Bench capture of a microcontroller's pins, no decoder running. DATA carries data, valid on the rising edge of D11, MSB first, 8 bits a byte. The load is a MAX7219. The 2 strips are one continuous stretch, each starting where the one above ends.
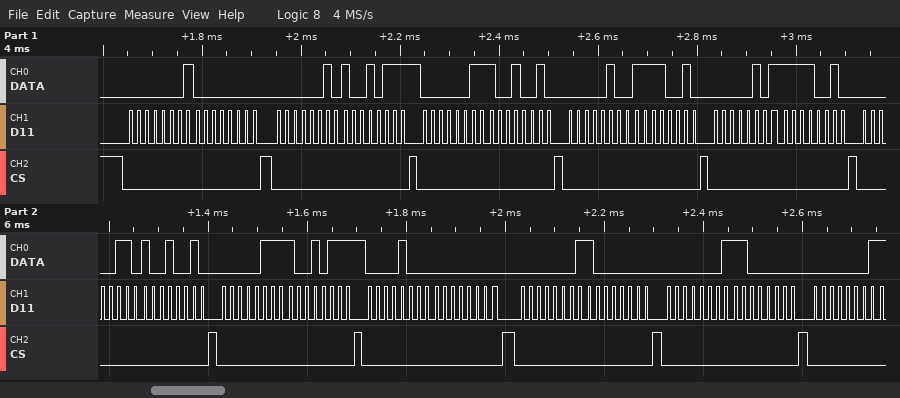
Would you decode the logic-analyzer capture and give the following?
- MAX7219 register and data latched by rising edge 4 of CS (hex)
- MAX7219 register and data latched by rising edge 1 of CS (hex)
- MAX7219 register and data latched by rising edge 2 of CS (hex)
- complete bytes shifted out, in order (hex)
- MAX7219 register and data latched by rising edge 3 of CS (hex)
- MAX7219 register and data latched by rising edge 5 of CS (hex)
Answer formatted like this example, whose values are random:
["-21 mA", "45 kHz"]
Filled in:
["register 0x4, data 0xF2", "register 0x1, data 0x00", "register 0x2, data 0x97", "0x01 0x00 0x02 0x97 0x03 0x92 0x04 0xF2 0x05 0xF2 0x06 0x92 0x07 0x97 0x08 0x00 0x01 0x80 0x01 0xC0 0x01", "register 0x3, data 0x92", "register 0x5, data 0xF2"]
